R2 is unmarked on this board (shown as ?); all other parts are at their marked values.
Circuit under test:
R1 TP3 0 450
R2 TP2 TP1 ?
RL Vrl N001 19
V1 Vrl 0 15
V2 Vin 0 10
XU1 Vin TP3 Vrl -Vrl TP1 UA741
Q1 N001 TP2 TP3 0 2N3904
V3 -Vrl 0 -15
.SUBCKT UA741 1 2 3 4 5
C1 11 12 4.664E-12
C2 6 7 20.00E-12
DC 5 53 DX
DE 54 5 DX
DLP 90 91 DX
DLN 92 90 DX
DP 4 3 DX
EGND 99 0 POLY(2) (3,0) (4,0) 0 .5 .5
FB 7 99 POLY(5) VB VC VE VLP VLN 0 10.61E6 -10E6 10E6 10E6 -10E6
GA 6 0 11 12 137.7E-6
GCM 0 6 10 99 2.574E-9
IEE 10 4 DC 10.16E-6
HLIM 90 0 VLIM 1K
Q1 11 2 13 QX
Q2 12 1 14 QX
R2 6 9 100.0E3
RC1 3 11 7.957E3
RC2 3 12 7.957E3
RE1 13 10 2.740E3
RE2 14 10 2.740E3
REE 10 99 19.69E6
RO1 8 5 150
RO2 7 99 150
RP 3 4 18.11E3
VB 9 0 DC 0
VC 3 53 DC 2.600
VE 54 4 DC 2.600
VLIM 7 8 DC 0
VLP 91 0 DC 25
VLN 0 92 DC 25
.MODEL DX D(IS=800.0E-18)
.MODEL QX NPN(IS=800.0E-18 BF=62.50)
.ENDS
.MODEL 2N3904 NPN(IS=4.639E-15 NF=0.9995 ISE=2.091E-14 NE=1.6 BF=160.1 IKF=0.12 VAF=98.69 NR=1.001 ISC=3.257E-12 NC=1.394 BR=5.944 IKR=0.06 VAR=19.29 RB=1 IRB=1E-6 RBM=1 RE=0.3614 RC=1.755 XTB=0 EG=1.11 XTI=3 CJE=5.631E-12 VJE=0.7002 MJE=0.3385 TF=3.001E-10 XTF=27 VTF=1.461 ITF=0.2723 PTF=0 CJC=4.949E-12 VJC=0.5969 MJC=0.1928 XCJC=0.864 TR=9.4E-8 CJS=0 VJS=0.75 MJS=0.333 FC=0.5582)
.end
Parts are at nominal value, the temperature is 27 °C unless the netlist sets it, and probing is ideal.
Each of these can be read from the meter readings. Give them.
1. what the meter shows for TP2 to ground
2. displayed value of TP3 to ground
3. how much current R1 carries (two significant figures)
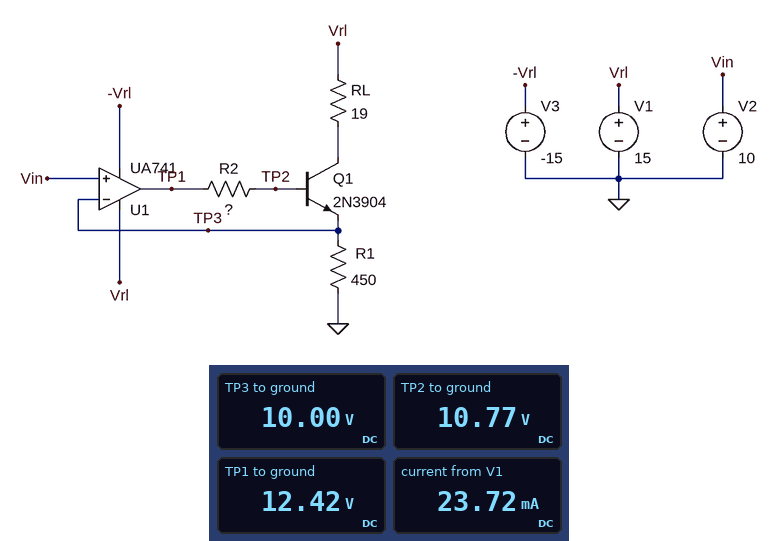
10.77 V
10.00 V
22 mA
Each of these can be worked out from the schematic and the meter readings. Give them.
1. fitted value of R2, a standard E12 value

10 kΩ
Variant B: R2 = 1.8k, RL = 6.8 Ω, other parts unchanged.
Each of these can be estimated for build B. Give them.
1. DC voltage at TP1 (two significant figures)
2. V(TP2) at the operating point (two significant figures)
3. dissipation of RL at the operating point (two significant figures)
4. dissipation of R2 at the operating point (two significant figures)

11 V
11 V
3.3 mW
49 µW
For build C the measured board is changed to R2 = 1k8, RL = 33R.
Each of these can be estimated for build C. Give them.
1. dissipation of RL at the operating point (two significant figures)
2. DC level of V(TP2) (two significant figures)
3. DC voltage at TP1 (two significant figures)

16 mW
11 V
11 V
